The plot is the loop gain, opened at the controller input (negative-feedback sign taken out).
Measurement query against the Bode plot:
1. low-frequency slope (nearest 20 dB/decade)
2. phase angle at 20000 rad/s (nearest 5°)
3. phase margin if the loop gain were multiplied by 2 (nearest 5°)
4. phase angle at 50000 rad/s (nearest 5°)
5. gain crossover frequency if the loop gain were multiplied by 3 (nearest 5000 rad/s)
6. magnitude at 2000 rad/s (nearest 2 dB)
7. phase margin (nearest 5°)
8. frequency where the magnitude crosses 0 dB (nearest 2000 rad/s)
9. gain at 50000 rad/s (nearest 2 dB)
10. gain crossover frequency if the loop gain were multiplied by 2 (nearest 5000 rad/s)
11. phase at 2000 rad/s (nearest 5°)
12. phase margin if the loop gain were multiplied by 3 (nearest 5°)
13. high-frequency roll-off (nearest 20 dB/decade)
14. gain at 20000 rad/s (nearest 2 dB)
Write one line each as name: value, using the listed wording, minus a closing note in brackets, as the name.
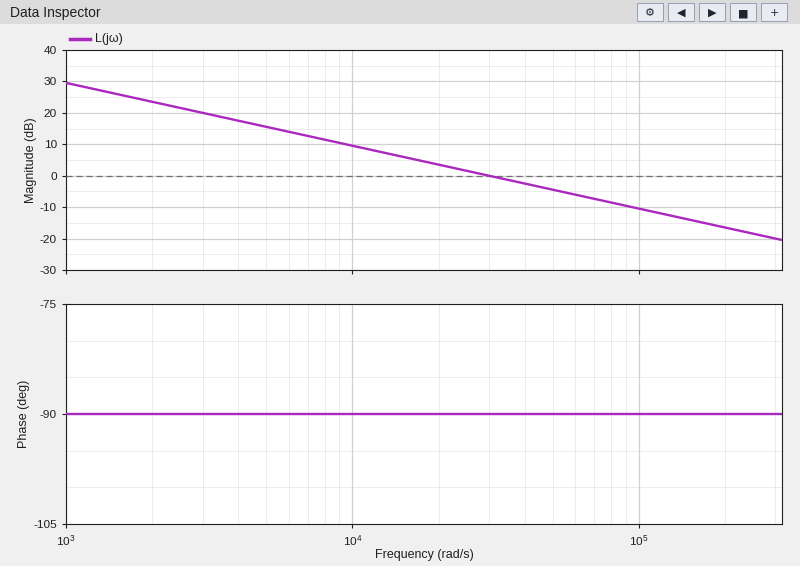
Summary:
low-frequency slope: -20 dB/decade
phase angle at 20000 rad/s: -90°
phase margin if the loop gain were multiplied by 2: 90°
phase angle at 50000 rad/s: -90°
gain crossover frequency if the loop gain were multiplied by 3: 90000 rad/s
magnitude at 2000 rad/s: 24 dB
phase margin: 90°
frequency where the magnitude crosses 0 dB: 30000 rad/s
gain at 50000 rad/s: -4 dB
gain crossover frequency if the loop gain were multiplied by 2: 60000 rad/s
phase at 2000 rad/s: -90°
phase margin if the loop gain were multiplied by 3: 90°
high-frequency roll-off: -20 dB/decade
gain at 20000 rad/s: 4 dB
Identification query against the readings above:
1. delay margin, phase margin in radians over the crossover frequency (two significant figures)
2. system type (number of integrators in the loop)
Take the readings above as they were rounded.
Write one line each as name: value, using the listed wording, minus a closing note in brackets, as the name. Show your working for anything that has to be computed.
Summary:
delay margin, phase margin in radians over the crossover frequency: 90 × π / 180 / 30000 = 0.000052 s
system type: 1
